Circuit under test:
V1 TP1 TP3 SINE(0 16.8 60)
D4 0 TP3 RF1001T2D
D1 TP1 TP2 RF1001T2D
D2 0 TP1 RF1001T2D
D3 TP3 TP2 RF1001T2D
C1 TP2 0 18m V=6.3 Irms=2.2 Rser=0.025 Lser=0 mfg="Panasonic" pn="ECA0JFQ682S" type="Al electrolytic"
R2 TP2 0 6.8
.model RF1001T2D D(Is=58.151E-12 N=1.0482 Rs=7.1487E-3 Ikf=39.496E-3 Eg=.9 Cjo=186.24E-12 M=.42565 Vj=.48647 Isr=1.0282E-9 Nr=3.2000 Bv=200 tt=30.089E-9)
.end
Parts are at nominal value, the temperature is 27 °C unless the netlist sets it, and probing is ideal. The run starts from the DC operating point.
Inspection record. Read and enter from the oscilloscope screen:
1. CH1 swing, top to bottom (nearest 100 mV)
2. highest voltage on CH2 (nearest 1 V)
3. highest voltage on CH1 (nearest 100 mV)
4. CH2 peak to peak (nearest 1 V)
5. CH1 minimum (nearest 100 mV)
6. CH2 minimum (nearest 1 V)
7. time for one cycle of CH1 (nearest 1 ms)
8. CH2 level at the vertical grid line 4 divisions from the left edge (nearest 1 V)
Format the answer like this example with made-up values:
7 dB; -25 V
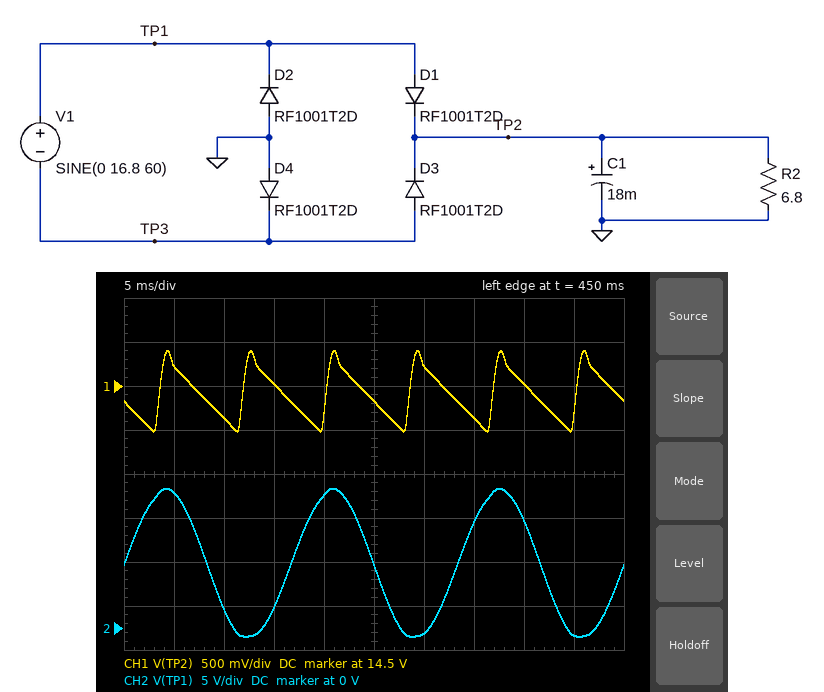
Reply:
900 mV; 16 V; 14.9 V; 17 V; 14.0 V; -1 V; 8 ms; 15 V
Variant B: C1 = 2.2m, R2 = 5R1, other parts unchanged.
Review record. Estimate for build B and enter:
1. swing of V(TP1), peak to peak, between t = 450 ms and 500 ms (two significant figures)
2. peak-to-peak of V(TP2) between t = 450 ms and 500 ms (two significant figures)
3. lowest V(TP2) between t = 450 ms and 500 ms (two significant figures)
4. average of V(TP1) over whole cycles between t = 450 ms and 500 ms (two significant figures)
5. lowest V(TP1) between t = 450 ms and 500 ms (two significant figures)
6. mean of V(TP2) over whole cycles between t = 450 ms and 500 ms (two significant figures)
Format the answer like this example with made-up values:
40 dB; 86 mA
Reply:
17 V; 5.9 V; 9.3 V; 6.2 V; -940 mV; 12 V
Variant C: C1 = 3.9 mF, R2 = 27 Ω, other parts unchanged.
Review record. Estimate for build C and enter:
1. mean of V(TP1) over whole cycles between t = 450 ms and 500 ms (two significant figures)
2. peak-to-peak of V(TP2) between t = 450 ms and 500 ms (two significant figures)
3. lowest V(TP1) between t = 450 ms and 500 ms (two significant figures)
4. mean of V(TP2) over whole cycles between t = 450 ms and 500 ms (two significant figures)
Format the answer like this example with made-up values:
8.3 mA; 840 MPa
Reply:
7.4 V; 970 mV; -860 mV; 15 V
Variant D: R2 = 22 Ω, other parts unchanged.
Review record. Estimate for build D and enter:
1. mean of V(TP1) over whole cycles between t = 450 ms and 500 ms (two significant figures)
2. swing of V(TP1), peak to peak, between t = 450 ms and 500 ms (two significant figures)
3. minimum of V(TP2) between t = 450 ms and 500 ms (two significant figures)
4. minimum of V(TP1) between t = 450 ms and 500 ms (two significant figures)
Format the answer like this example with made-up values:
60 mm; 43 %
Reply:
7.4 V; 17 V; 15 V; -880 mV
